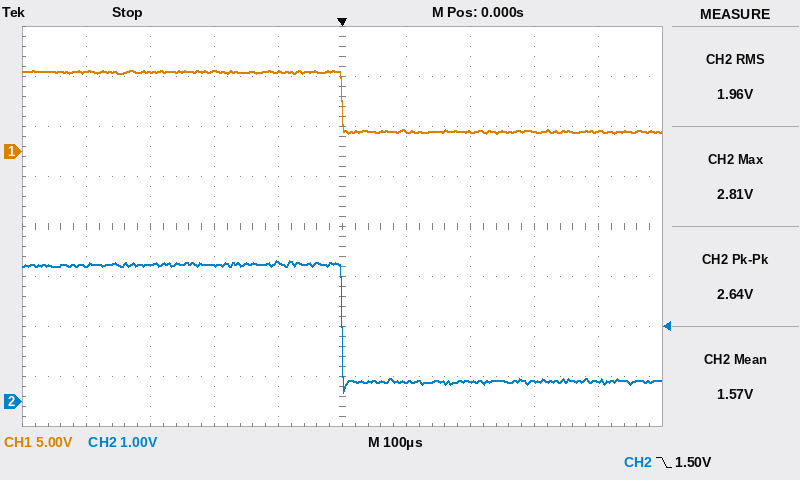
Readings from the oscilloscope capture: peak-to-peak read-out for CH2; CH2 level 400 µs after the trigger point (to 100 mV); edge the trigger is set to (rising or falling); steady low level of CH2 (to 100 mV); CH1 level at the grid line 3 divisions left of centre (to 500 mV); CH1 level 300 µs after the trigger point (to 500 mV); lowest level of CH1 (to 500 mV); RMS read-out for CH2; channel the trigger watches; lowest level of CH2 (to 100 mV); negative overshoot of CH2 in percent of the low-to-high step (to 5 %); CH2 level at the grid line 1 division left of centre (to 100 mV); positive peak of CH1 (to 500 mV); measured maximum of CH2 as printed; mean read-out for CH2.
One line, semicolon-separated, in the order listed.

2.64 V; 400 mV; falling; 400 mV; 8.0 V; 2.0 V; 2.0 V; 1.96 V; CH2; 200 mV; 10 %; 2.8 V; 8.0 V; 2.81 V; 1.57 V
